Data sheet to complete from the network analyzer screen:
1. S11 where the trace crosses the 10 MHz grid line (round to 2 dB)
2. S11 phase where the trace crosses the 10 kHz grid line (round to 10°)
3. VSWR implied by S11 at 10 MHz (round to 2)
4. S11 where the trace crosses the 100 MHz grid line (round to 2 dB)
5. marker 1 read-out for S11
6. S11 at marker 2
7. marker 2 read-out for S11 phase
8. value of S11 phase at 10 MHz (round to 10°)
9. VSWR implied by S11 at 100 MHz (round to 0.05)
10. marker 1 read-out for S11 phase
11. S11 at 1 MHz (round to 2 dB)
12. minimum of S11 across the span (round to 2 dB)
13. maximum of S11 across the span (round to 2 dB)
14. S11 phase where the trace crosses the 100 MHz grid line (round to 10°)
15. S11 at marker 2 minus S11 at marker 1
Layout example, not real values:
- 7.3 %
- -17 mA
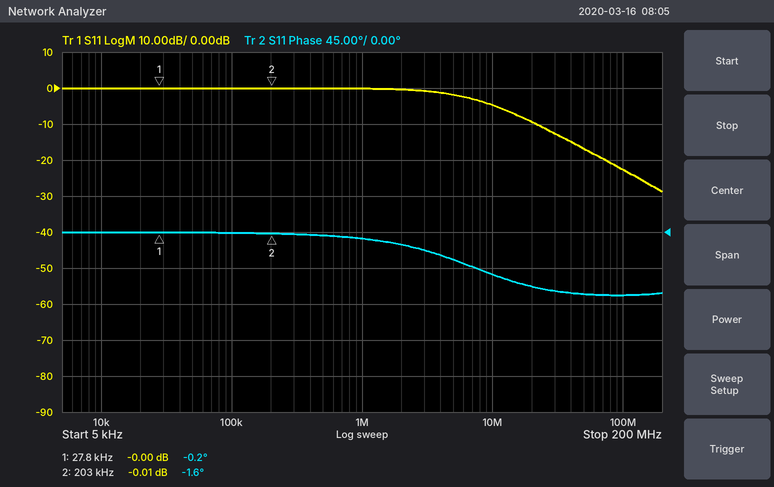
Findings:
- -4 dB
- 0°
- 4
- -22 dB
- -0.00 dB
- -0.01 dB
- -1.6°
- -50°
- 1.15
- -0.2°
- 0 dB
- -28 dB
- 0 dB
- -80°
- -0.01 dB
